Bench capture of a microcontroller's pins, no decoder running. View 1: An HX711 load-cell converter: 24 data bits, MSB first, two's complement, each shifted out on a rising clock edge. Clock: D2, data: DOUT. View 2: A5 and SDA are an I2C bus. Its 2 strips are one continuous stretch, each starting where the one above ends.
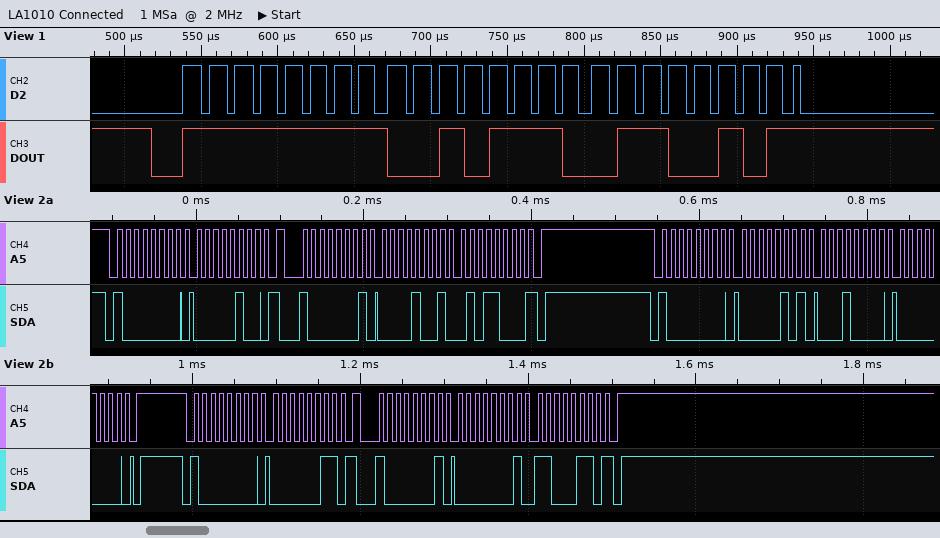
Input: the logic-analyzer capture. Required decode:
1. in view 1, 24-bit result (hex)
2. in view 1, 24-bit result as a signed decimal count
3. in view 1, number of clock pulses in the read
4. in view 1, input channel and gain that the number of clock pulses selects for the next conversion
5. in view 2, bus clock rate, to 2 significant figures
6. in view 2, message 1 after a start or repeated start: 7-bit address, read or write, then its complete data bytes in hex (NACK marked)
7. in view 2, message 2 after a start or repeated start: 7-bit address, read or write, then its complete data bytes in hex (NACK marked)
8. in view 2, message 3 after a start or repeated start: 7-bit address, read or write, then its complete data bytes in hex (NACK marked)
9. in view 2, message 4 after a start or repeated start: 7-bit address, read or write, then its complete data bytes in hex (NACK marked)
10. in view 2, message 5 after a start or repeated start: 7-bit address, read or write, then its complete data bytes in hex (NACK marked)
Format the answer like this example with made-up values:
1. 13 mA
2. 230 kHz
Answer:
1. 0xFF2E65
2. -53659
3. 25
4. channel A, gain 128
5. 100 kHz
6. 0x40 write: 04
7. 0x40 read: 09 58 NACK
8. 0x40 write: 05 10 00
9. 0x40 write: 03
10. 0x40 read: 01 C6 NACK
